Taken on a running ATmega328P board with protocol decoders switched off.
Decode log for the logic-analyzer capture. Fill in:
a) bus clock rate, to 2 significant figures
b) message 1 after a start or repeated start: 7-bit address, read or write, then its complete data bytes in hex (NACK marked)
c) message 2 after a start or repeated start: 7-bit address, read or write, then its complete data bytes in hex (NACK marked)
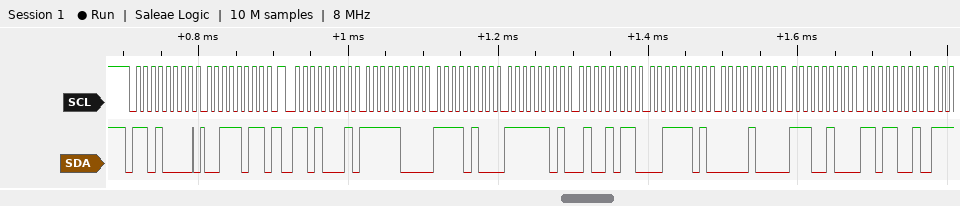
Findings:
100 kHz
0x68 write: 3B
0x68 read: F8 F4 FD 4B 3D 08 E4 D9
